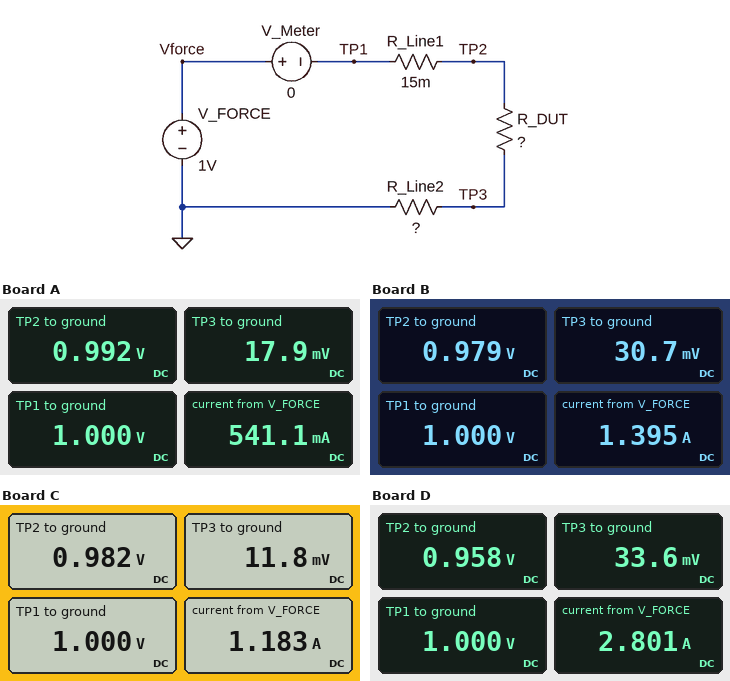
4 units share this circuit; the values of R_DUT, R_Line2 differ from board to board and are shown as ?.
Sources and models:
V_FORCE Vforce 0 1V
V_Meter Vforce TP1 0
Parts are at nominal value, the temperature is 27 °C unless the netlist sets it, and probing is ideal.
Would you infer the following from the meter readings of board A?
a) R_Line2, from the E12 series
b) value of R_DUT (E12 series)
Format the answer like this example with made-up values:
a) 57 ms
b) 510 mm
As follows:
a) 0.033 Ω
b) 1.8 Ω
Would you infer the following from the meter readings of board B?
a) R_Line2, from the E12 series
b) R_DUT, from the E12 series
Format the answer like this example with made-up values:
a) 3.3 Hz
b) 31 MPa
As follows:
a) 0.022 Ω
b) 0.68 Ω
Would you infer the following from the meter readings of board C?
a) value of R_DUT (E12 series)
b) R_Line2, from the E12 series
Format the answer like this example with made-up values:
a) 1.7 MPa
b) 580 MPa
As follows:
a) 0.82 Ω
b) 0.01 Ω
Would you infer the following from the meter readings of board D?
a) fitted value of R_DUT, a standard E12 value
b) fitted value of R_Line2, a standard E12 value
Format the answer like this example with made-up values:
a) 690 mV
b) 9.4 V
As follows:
a) 0.33 Ω
b) 0.012 Ω
